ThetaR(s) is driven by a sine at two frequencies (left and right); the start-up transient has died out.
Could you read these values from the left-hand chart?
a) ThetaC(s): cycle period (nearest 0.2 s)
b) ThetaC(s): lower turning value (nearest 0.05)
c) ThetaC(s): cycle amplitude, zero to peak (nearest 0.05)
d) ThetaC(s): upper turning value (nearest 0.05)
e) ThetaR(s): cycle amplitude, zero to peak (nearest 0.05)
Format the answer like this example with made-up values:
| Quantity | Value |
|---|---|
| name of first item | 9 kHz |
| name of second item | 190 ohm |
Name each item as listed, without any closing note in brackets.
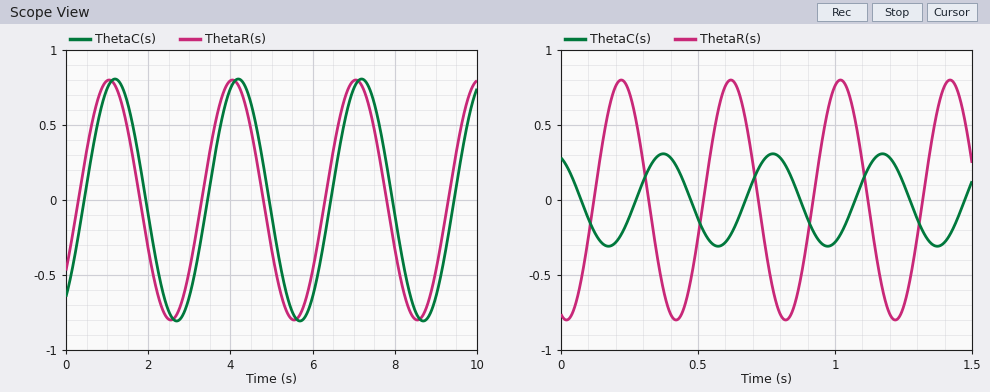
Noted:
| Quantity | Value |
|---|---|
| ThetaC(s): cycle period | 3.0 s |
| ThetaC(s): lower turning value | -0.80 |
| ThetaC(s): cycle amplitude, zero to peak | 0.80 |
| ThetaC(s): upper turning value | 0.80 |
| ThetaR(s): cycle amplitude, zero to peak | 0.80 |
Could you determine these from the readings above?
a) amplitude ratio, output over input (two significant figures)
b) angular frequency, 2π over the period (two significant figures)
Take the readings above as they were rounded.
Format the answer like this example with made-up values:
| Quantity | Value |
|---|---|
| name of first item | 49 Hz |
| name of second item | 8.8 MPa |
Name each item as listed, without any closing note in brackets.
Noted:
| Quantity | Value |
|---|---|
| amplitude ratio, output over input | 1.0 |
| angular frequency, 2π over the period | 2.1 rad/s |
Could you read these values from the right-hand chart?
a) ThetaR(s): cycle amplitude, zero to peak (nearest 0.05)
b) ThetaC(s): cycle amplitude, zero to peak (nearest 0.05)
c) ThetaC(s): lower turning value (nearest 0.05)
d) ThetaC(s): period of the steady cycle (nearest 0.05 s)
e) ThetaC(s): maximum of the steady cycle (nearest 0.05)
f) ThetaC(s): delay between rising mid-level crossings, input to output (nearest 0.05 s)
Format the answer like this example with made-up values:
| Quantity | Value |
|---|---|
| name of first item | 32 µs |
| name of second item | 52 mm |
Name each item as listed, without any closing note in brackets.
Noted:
| Quantity | Value |
|---|---|
| ThetaR(s): cycle amplitude, zero to peak | 0.80 |
| ThetaC(s): cycle amplitude, zero to peak | 0.30 |
| ThetaC(s): lower turning value | -0.30 |
| ThetaC(s): period of the steady cycle | 0.40 s |
| ThetaC(s): maximum of the steady cycle | 0.30 |
| ThetaC(s): delay between rising mid-level crossings, input to output | 0.15 s |
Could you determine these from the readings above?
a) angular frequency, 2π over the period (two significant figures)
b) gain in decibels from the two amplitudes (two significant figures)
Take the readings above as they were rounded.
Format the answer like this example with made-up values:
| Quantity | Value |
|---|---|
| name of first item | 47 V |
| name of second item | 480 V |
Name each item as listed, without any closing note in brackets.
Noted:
| Quantity | Value |
|---|---|
| angular frequency, 2π over the period | 16 rad/s |
| gain in decibels from the two amplitudes | -8.5 dB |
